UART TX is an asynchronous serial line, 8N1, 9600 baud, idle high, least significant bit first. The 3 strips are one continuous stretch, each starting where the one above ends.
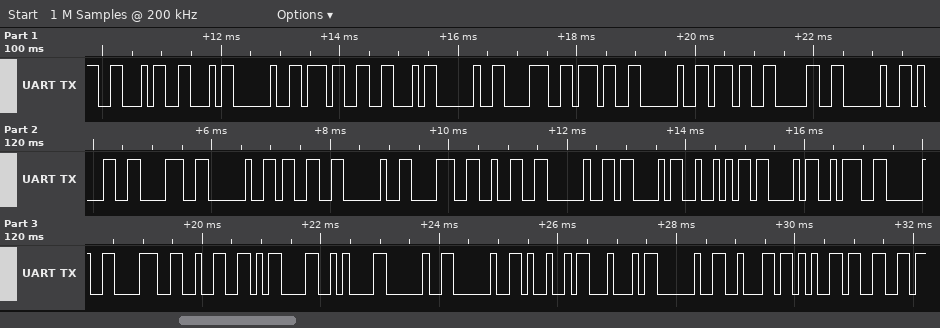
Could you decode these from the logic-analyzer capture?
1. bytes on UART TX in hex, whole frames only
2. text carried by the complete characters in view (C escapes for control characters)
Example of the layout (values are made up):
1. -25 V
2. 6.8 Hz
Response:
1. 46 46 20 37 46 20 38 37 20 37 30 20 31 38 20 33 20 38 32 20 43 52 43 3A 20 38 32 0D 0A 20 20 49 44 20 62 65 66
2. "FF 7F 87 70 18 3 82 CRC: 82\r\n  ID bef"
